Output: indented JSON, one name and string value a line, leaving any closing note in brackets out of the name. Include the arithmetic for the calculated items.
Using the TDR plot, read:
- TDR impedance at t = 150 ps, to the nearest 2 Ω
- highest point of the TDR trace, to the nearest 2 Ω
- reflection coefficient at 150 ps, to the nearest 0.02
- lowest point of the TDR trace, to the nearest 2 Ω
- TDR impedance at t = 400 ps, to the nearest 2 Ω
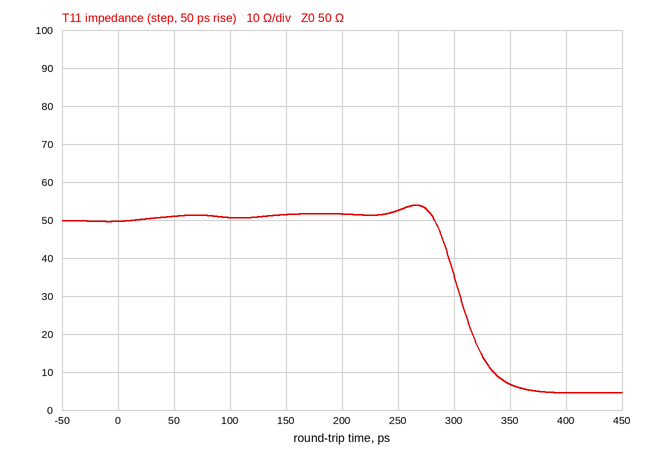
{
  "TDR impedance at t = 150 ps, to the nearest 2 Ω": "52 Ω",
  "highest point of the TDR trace, to the nearest 2 Ω": "54 Ω",
  "reflection coefficient at 150 ps, to the nearest 0.02": "(52 − 50)/(52 + 50) ≈ +0.02",
  "lowest point of the TDR trace, to the nearest 2 Ω": "4 Ω",
  "TDR impedance at t = 400 ps, to the nearest 2 Ω": "4 Ω"
}
